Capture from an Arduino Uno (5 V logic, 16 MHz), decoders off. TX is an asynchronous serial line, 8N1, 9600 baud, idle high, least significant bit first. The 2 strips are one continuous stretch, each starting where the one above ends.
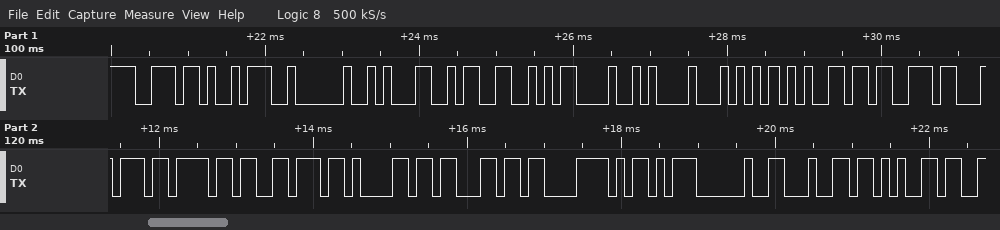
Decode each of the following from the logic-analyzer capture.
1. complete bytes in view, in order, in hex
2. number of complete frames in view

0x6E 0x3A 0x20 0x31 0x33 0x0D 0x0A 0x54 0x65 0x73 0x74 0x6F 0x76 0x61 0x63 0xC3 0xAD 0x20 0x64 0x65
20
